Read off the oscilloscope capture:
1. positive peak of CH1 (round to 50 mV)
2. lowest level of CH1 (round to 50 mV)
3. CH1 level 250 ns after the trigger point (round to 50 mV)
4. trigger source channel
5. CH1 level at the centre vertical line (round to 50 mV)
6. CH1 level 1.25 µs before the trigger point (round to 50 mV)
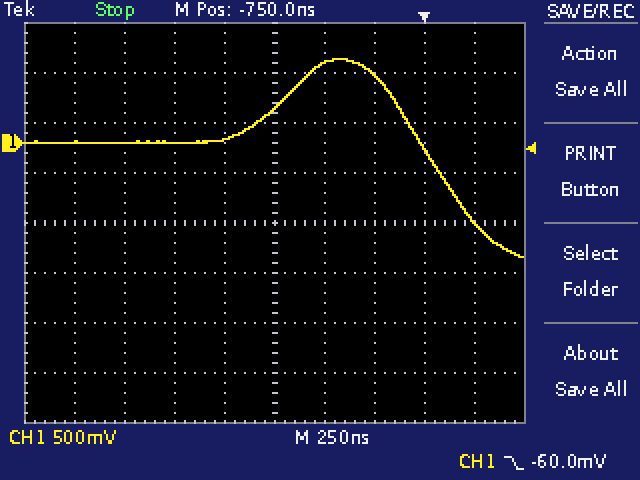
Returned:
850 mV
-1.15 V
-800 mV
CH1
350 mV
0 mV
